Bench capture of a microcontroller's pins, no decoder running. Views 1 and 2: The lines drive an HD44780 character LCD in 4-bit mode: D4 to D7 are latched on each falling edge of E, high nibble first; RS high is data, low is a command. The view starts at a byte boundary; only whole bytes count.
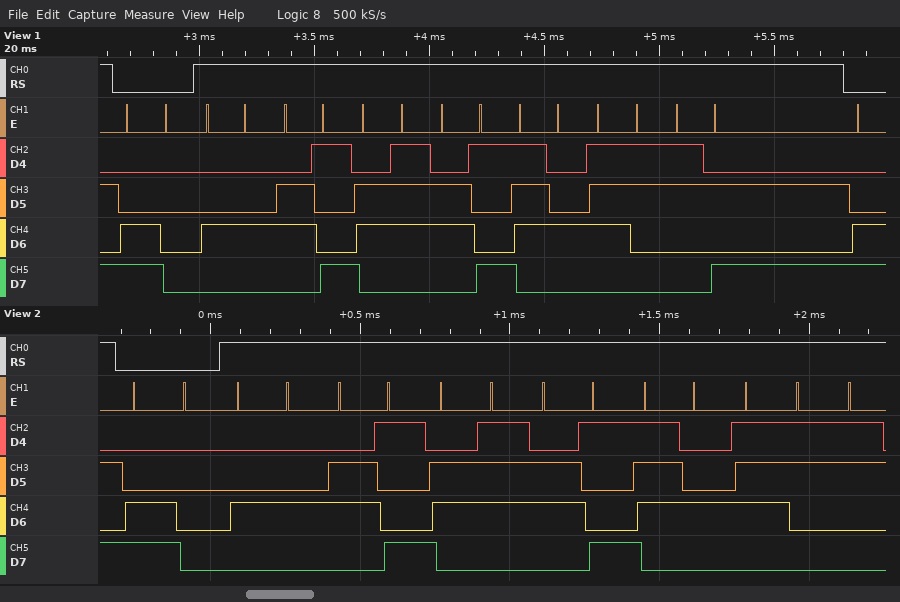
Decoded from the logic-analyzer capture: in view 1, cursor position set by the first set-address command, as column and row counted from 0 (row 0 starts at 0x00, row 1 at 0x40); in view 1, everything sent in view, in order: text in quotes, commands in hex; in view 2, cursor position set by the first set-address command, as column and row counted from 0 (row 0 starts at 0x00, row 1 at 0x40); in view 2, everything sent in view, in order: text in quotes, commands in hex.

column 0, row 1
0xC0 "Digits:"
column 0, row 1
0xC0 "Digits"
